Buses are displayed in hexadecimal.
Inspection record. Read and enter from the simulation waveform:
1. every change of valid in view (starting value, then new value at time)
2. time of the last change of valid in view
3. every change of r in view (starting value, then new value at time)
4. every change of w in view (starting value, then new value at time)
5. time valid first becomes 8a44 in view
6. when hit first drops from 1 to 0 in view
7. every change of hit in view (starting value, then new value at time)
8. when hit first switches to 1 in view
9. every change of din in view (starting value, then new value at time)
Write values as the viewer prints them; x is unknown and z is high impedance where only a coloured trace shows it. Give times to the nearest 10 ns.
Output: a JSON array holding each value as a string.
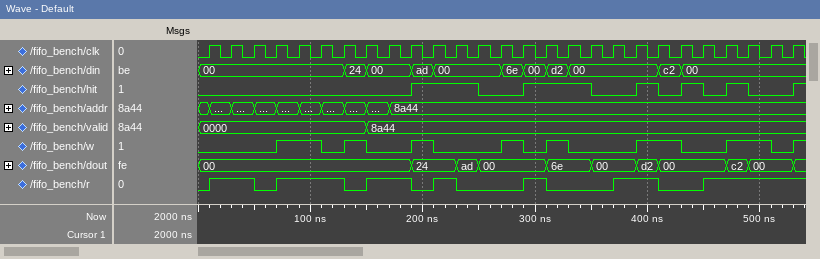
["0000, 8a44 at 150 ns", "150 ns", "0, 1 at 10 ns, 0 at 50 ns, 1 at 70 ns, 0 at 130 ns, 1 at 150 ns, 0 at 190 ns, 1 at 210 ns, 0 at 230 ns, 1 at 290 ns, 0 at 310 ns, 1 at 370 ns, 0 at 410 ns, 1 at 450 ns", "0, 1 at 70 ns, 0 at 110 ns, 1 at 130 ns, 0 at 150 ns, 1 at 190 ns, 0 at 210 ns, 1 at 270 ns, 0 at 290 ns, 1 at 310 ns, 0 at 330 ns, 1 at 390 ns, 0 at 430 ns, 1 at 470 ns, 0 at 510 ns, 1 at 530 ns", "150 ns", "250 ns", "0, 1 at 190 ns, 0 at 250 ns, 1 at 290 ns, 0 at 350 ns, 1 at 390 ns, 0 at 410 ns, 1 at 430 ns, 0 at 450 ns, 1 at 470 ns, 0 at 490 ns, 1 at 530 ns", "190 ns", "00, 24 at 130 ns, 00 at 150 ns, ad at 190 ns, 00 at 210 ns, 6e at 270 ns, 00 at 290 ns, d2 at 310 ns, 00 at 330 ns, c2 at 410 ns, 00 at 430 ns"]
